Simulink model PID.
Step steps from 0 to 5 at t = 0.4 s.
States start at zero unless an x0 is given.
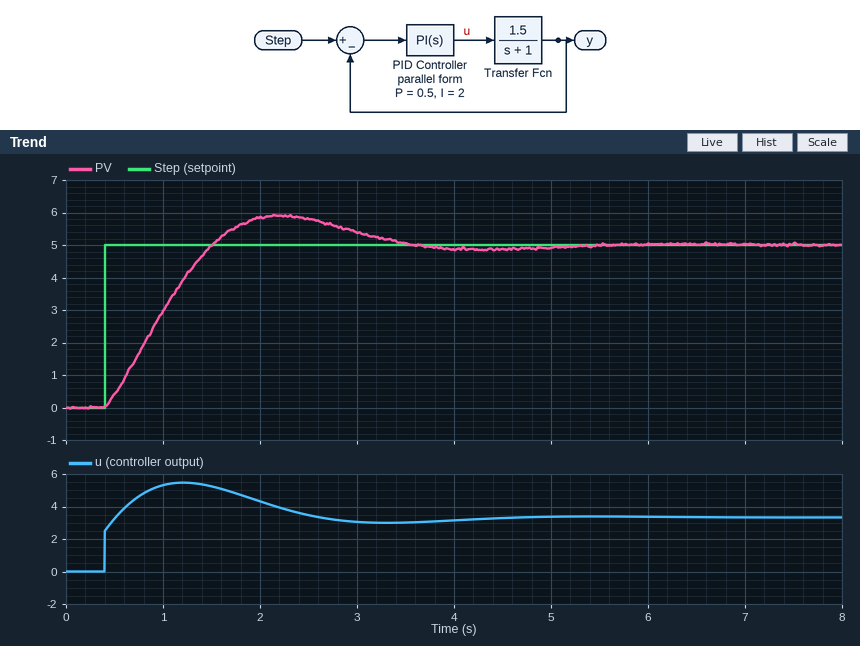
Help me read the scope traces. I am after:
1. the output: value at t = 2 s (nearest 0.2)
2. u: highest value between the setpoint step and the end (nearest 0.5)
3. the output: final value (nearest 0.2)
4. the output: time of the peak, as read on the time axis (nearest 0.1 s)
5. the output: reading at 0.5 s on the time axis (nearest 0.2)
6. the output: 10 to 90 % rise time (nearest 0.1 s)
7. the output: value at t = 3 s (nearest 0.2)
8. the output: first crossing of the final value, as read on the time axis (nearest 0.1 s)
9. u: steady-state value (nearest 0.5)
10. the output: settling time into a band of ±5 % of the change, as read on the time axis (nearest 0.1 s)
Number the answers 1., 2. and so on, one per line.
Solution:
1. 5.8
2. 5.5
3. 5.0
4. 2.2 s
5. 0.4
6. 0.8 s
7. 5.4
8. 1.5 s
9. 3.5
10. 3.2 s
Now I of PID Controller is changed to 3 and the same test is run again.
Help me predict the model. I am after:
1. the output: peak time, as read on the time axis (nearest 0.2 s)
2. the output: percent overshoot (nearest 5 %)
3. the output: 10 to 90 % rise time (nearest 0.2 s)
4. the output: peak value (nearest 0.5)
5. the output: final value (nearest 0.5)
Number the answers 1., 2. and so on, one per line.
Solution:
1. 1.8 s
2. 25 %
3. 0.6 s
4. 6.5
5. 5.0
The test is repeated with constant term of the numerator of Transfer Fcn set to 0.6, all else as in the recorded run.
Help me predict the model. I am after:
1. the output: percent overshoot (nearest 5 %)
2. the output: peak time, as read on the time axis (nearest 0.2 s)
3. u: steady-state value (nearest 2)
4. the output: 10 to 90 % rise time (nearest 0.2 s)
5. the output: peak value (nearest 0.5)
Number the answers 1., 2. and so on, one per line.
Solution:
1. 10 %
2. 3.6 s
3. 8
4. 1.6 s
5. 5.5
